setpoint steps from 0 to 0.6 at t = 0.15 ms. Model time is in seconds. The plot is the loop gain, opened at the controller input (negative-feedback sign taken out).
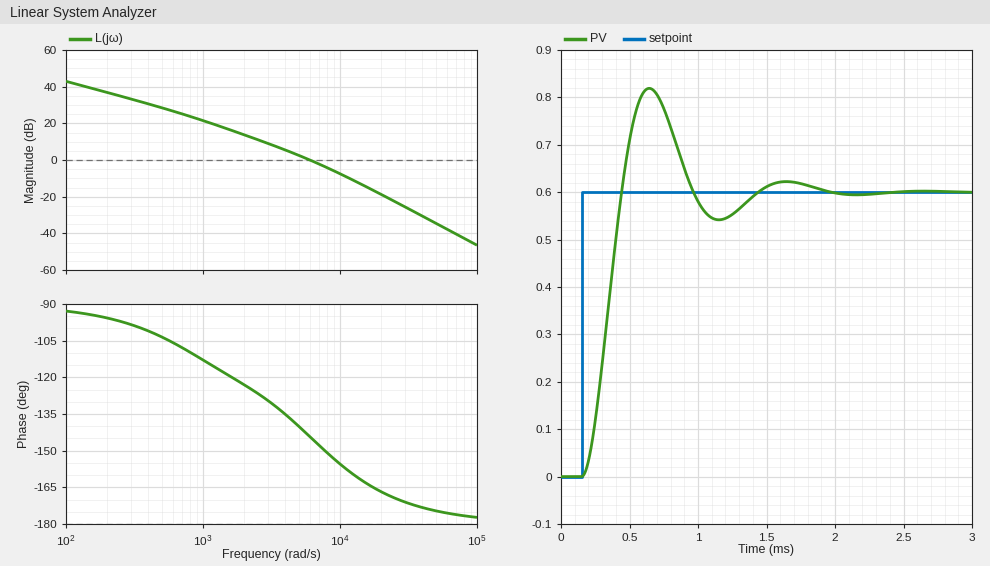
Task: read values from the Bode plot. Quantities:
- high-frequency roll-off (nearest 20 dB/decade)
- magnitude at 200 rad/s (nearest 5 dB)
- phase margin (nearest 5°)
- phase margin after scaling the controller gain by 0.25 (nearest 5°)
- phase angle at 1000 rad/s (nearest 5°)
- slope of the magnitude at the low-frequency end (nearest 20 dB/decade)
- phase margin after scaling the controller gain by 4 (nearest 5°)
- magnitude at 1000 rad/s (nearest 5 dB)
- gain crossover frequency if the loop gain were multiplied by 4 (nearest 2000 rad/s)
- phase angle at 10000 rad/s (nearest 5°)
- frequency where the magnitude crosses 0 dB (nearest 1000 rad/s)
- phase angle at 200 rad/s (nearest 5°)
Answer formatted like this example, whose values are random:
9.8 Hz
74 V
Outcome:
-40 dB/decade
35 dB
35°
55°
-115°
-20 dB/decade
20°
20 dB
14000 rad/s
-155°
6000 rad/s
-95°
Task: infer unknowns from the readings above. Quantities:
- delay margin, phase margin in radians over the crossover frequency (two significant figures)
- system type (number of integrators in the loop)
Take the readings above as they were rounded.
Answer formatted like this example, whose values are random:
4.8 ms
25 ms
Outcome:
0.00010 s
1
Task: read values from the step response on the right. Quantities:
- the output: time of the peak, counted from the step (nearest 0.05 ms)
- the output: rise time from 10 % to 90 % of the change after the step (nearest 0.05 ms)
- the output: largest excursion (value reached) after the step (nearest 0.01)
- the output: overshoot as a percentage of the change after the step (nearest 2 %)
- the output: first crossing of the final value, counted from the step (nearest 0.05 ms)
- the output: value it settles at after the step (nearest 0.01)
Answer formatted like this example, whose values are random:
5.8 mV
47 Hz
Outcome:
0.50 ms
0.20 ms
0.82
36 %
0.30 ms
0.60
